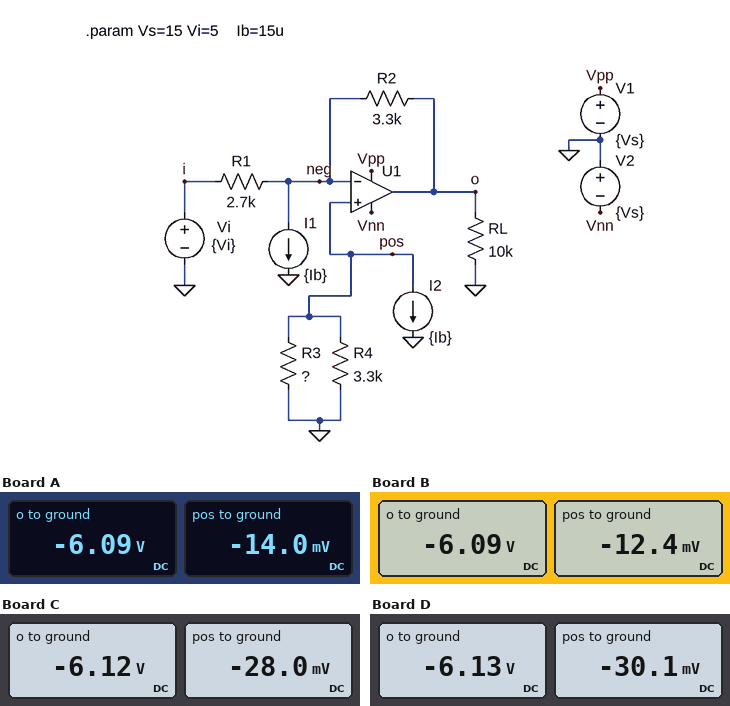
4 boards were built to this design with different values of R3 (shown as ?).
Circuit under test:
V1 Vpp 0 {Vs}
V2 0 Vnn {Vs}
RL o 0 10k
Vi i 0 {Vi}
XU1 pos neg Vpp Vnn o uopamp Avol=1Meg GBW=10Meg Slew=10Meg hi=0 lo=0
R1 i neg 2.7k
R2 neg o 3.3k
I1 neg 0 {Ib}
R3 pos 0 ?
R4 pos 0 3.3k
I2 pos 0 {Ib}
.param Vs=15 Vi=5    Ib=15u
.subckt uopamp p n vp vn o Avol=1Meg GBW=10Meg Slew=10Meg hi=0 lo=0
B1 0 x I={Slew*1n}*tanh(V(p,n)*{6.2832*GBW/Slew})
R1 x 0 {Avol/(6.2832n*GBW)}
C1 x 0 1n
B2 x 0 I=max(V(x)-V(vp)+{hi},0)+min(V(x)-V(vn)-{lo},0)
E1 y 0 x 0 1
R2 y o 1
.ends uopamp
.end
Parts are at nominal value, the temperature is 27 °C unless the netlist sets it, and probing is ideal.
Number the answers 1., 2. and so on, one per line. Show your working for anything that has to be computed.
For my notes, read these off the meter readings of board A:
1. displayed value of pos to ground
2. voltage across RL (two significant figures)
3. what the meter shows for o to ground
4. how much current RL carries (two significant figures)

1. -14.0 mV
2. 0 V - (-6.09 V) = 6.1 V
3. -6.09 V
4. (0 V - (-6.09 V)) / 10 kΩ = 610 µA
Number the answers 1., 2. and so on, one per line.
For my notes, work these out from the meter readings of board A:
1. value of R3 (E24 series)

1. 1.3 kΩ
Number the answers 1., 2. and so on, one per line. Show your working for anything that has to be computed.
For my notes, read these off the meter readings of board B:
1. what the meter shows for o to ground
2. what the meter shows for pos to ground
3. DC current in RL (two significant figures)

1. -6.09 V
2. -12.4 mV
3. (0 V - (-6.09 V)) / 10 kΩ = 610 µA
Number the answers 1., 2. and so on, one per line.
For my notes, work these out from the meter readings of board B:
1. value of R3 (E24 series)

1. 1.1 kΩ
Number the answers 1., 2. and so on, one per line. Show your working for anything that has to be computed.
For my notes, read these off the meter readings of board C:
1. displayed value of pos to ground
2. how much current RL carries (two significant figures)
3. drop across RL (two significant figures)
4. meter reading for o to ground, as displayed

1. -28.0 mV
2. (0 V - (-6.12 V)) / 10 kΩ = 610 µA
3. 0 V - (-6.12 V) = 6.1 V
4. -6.12 V
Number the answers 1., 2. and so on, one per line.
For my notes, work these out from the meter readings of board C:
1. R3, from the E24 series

1. 4.3 kΩ
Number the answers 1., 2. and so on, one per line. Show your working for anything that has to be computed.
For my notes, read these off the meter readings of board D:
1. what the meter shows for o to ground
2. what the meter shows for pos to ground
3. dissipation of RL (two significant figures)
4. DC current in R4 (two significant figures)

1. -6.13 V
2. -30.1 mV
3. (0 V - (-6.13 V))^2 / 10 kΩ = 3.8 mW
4. (0 V - (-30.1 mV)) / 3.3 kΩ = 9.1 µA
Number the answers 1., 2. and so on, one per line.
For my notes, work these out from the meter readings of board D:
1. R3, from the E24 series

1. 5.1 kΩ
